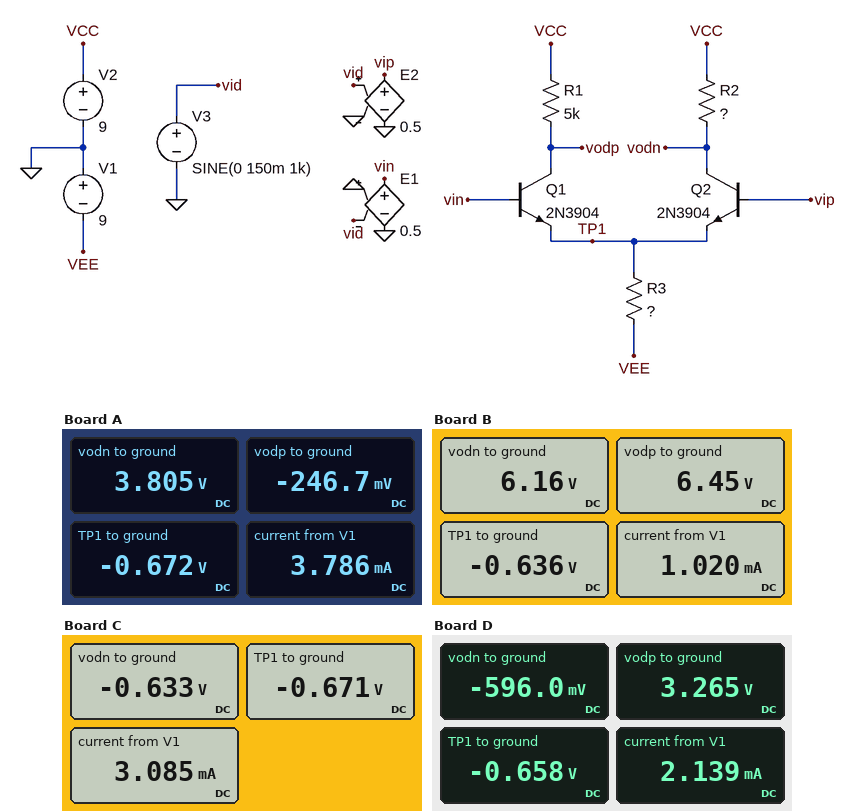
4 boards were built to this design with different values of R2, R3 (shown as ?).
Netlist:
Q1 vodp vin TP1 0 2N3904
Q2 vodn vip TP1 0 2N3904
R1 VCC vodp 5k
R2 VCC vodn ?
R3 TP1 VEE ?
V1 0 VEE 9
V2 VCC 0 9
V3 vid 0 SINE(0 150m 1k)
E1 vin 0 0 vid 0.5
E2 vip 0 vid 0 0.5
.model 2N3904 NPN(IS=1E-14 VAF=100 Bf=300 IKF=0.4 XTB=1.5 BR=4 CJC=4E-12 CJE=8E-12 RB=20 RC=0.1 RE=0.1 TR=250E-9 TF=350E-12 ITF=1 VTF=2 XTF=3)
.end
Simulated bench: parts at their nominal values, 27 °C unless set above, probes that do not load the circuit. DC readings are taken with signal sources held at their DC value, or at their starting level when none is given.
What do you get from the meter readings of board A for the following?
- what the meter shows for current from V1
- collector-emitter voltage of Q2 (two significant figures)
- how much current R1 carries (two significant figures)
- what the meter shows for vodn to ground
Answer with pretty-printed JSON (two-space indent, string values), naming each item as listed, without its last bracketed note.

{
  "what the meter shows for current from V1": "3.786 mA",
  "collector-emitter voltage of Q2": "4.5 V",
  "how much current R1 carries": "1.8 mA",
  "what the meter shows for vodn to ground": "3.805 V"
}
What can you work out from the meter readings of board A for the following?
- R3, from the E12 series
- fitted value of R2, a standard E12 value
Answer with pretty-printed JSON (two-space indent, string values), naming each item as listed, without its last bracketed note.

{
  "R3, from the E12 series": "2.2 kΩ",
  "fitted value of R2, a standard E12 value": "2.7 kΩ"
}
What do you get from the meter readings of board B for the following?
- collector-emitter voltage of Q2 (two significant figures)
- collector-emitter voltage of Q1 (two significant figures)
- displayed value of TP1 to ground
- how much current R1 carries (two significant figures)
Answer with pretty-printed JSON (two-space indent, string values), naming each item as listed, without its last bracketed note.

{
  "collector-emitter voltage of Q2": "6.8 V",
  "collector-emitter voltage of Q1": "7.1 V",
  "displayed value of TP1 to ground": "-0.636 V",
  "how much current R1 carries": "510 µA"
}
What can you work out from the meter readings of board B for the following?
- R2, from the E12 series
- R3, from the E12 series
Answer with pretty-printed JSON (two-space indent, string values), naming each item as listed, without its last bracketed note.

{
  "R2, from the E12 series": "5.6 kΩ",
  "R3, from the E12 series": "8.2 kΩ"
}
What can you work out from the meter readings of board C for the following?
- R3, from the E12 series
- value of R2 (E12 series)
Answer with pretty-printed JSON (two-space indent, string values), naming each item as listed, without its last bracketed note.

{
  "R3, from the E12 series": "2.7 kΩ",
  "value of R2": "8.2 kΩ"
}
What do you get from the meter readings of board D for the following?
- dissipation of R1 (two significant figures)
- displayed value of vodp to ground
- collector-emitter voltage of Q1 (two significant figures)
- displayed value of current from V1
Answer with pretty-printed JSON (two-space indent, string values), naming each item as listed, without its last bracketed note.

{
  "dissipation of R1": "6.6 mW",
  "displayed value of vodp to ground": "3.265 V",
  "collector-emitter voltage of Q1": "3.9 V",
  "displayed value of current from V1": "2.139 mA"
}
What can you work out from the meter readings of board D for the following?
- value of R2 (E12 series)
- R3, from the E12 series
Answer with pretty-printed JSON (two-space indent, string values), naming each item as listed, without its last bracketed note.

{
  "value of R2": "10 kΩ",
  "R3, from the E12 series": "3.9 kΩ"
}
